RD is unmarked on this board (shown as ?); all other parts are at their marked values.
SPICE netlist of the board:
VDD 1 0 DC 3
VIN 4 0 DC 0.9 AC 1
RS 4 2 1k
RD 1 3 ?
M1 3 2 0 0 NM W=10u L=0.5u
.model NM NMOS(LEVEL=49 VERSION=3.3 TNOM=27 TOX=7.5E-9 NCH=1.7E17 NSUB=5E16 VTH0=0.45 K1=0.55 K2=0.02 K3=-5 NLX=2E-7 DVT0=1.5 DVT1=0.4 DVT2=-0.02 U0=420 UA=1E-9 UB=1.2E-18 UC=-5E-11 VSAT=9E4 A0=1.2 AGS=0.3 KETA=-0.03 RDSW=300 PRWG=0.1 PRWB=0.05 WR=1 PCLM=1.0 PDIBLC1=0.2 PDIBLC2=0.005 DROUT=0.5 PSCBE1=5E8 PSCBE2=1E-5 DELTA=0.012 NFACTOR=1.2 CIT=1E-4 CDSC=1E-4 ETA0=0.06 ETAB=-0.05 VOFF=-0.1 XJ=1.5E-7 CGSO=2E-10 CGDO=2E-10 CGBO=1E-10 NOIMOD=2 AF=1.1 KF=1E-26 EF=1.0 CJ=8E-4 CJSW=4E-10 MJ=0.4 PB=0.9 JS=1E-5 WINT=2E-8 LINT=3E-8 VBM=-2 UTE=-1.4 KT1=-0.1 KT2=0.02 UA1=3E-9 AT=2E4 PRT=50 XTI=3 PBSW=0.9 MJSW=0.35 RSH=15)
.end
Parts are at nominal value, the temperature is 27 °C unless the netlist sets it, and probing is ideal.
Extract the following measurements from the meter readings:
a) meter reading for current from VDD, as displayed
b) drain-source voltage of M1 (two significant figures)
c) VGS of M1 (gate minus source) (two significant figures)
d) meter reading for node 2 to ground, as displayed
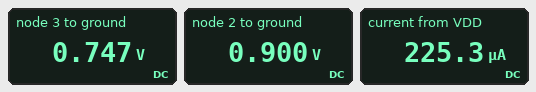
225.3 µA
750 mV
900 mV
0.900 V
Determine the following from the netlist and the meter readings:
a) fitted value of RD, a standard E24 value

10 kΩ
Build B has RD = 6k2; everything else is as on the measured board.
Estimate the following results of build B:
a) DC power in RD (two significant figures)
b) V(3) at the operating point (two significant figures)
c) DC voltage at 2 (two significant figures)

370 µW
1.5 V
900 mV
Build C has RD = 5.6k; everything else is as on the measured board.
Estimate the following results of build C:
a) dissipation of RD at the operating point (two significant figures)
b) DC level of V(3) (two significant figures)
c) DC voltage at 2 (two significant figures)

340 µW
1.6 V
900 mV
